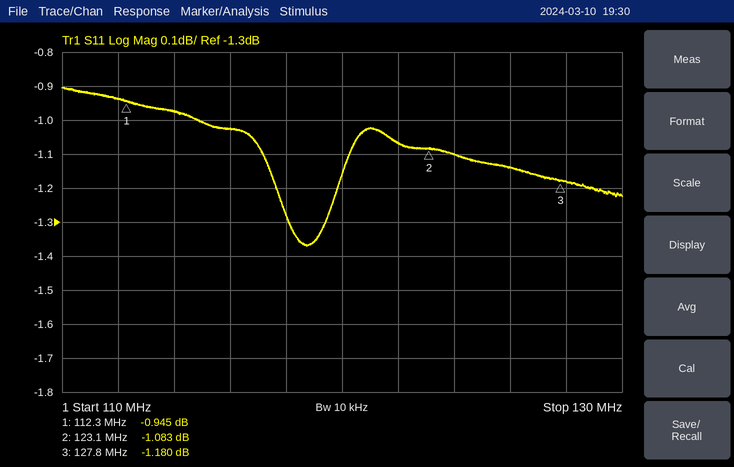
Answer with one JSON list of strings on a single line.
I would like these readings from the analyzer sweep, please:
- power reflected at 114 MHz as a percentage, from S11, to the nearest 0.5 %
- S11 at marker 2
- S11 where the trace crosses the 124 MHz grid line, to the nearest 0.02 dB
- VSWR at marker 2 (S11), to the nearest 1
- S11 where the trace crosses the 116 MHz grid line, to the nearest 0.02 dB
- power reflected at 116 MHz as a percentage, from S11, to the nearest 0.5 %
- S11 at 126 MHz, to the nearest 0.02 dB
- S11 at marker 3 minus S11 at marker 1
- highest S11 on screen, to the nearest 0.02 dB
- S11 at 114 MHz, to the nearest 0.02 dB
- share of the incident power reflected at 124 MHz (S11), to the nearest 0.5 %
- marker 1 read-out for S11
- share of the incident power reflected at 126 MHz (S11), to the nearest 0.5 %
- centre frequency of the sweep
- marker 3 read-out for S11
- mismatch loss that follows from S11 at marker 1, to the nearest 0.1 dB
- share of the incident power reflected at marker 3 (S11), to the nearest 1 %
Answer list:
["80.0 %", "-1.083 dB", "-1.10 dB", "16", "-1.02 dB", "79.0 %", "-1.14 dB", "-0.235 dB", "-0.90 dB", "-0.98 dB", "77.5 %", "-0.945 dB", "77.0 %", "120 MHz", "-1.180 dB", "7.1 dB", "76 %"]
